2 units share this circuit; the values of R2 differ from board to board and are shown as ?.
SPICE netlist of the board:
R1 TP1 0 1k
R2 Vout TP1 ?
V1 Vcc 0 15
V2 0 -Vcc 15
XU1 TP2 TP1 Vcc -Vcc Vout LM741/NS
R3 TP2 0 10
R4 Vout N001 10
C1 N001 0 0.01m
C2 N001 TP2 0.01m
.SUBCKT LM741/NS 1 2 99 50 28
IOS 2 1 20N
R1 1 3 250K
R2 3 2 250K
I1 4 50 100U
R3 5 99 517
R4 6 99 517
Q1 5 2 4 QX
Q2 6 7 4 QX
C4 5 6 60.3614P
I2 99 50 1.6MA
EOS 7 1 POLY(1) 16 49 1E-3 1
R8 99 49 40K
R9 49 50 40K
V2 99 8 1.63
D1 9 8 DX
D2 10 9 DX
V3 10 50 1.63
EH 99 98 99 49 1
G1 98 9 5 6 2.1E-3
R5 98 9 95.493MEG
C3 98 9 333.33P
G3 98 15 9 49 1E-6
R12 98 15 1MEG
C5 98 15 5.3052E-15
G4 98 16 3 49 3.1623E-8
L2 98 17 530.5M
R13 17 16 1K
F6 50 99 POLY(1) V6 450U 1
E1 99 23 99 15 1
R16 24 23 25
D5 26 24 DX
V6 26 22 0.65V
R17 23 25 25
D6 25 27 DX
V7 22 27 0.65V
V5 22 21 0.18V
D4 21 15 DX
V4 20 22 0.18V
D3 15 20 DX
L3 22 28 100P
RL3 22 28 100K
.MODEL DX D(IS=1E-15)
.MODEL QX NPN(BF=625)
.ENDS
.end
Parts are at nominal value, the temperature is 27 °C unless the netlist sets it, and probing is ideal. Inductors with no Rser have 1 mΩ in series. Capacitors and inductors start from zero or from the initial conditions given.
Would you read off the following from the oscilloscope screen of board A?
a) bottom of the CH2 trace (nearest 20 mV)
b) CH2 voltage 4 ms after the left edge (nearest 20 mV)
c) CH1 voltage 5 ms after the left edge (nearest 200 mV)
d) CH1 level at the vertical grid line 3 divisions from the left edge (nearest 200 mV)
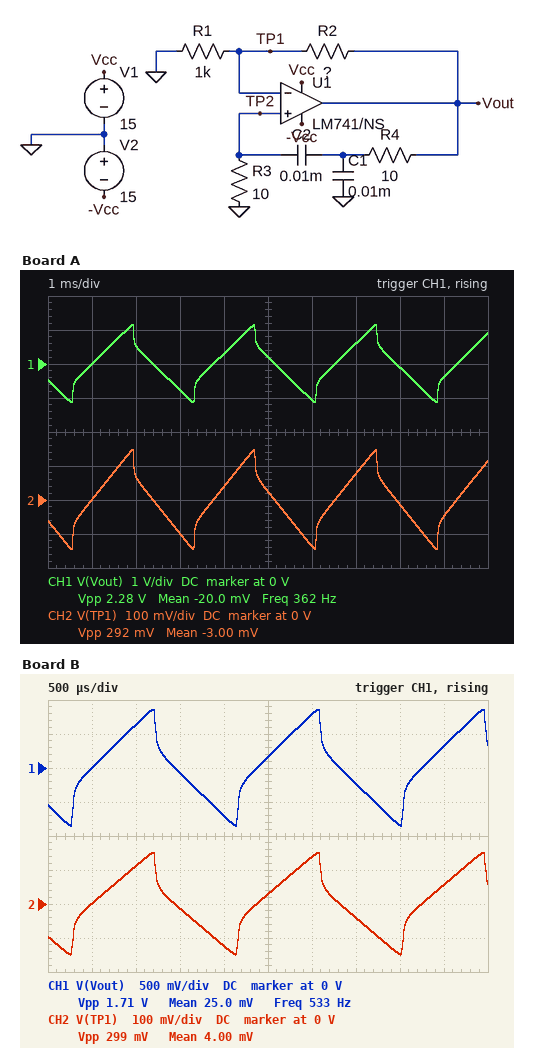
-140 mV
40 mV
200 mV
-800 mV
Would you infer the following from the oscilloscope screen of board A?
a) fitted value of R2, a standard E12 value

6.8 kΩ
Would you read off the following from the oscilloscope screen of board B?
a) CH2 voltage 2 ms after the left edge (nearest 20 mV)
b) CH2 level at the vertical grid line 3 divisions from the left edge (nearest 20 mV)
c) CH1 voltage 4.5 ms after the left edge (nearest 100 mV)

-120 mV
-20 mV
300 mV
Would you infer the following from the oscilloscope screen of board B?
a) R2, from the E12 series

4.7 kΩ
